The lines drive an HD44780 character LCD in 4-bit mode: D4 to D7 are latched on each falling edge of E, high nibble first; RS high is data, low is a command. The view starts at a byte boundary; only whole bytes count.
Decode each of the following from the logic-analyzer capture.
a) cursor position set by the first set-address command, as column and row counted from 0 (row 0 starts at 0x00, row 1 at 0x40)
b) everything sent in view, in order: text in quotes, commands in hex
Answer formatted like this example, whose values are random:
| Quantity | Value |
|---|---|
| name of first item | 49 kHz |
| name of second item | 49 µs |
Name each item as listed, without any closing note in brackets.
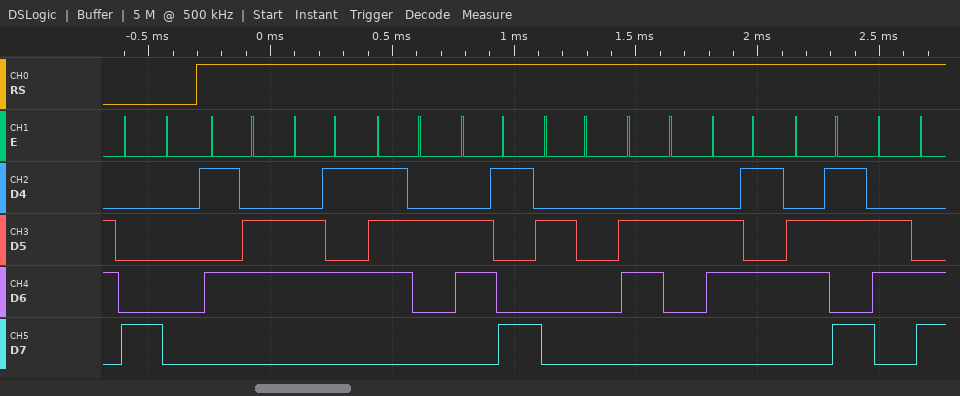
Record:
| Quantity | Value |
|---|---|
| cursor position set by the first set-address command, as column and row counted from 0 | column 0, row 0 |
| everything sent in view, in order: text in quotes, commands in hex | 0x80 "Veri bekl" |
